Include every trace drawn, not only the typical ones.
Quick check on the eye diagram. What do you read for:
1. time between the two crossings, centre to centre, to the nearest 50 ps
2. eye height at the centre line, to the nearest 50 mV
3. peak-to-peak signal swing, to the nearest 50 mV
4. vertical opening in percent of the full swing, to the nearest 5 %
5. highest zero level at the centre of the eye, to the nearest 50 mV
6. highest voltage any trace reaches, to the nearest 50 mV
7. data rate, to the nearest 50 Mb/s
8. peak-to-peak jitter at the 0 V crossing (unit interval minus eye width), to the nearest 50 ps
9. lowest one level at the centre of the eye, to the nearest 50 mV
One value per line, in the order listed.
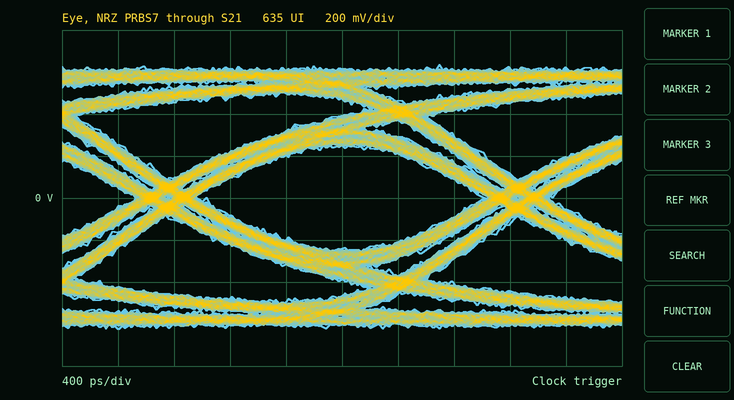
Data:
2.50 ns
500 mV
1.25 V
40 %
-250 mV
650 mV
400 Mb/s
500 ps
250 mV
